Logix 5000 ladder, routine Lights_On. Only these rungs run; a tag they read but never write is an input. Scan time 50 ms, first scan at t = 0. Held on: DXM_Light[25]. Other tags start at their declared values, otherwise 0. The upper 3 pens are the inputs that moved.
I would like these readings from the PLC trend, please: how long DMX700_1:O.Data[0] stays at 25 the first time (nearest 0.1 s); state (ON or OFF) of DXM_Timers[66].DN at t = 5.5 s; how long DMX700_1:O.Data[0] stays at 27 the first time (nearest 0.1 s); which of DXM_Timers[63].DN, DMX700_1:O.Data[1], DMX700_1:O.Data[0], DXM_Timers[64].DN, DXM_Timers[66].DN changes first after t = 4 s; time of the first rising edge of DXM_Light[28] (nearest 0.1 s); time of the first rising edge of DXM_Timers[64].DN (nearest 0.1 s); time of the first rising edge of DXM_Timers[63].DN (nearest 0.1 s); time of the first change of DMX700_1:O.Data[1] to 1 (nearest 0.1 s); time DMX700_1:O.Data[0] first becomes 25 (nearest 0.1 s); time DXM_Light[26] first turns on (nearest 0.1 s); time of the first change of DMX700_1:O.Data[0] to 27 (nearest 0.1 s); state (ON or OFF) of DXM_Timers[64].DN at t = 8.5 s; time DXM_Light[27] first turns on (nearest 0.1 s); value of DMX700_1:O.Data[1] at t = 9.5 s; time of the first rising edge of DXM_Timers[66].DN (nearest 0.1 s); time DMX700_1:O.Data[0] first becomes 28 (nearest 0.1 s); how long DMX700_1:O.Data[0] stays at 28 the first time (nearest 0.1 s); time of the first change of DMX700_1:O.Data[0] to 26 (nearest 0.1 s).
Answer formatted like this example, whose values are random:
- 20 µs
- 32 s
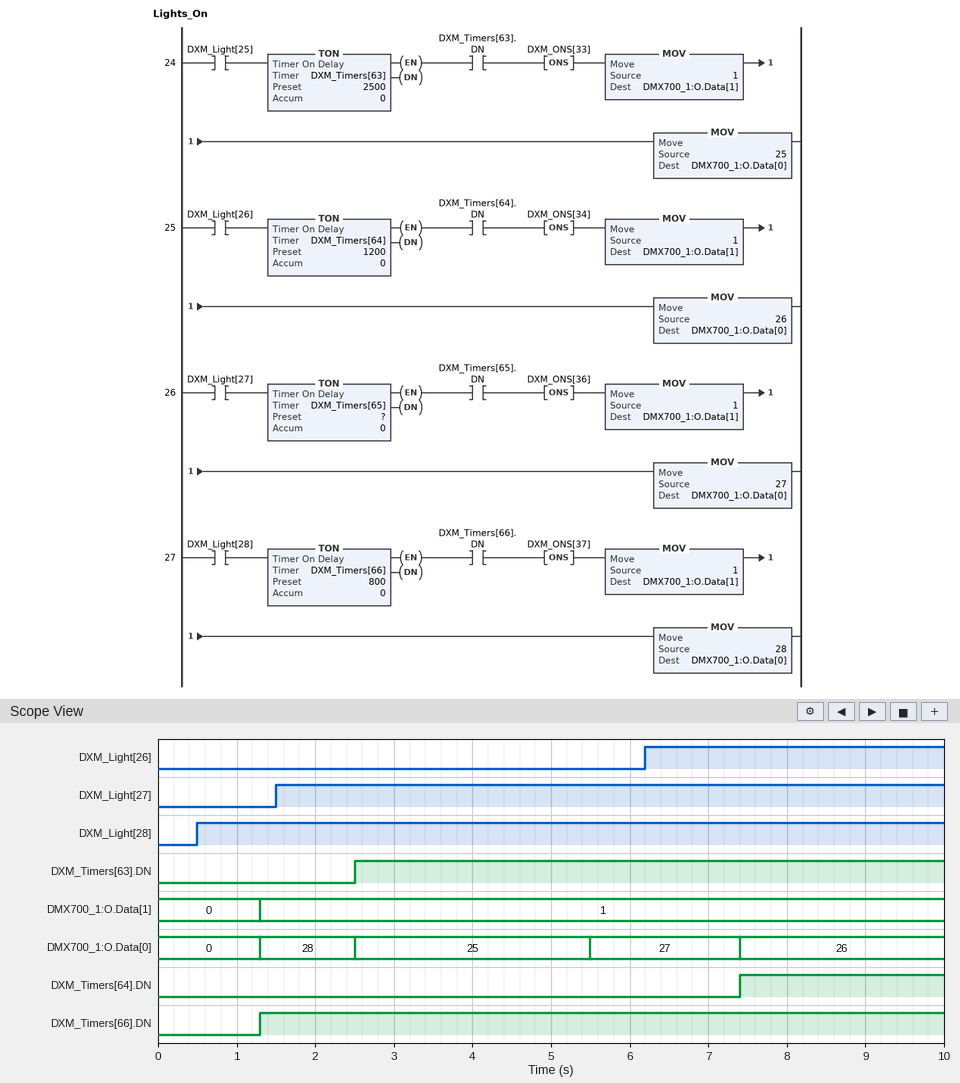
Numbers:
- 3.0 s
- ON
- 1.9 s
- DMX700_1:O.Data[0]
- 0.5 s
- 7.4 s
- 2.5 s
- 1.3 s
- 2.5 s
- 6.2 s
- 5.5 s
- ON
- 1.5 s
- 1
- 1.3 s
- 1.3 s
- 1.2 s
- 7.4 s
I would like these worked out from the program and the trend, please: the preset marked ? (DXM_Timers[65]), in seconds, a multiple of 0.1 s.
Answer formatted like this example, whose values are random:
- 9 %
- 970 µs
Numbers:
- 4.0 s
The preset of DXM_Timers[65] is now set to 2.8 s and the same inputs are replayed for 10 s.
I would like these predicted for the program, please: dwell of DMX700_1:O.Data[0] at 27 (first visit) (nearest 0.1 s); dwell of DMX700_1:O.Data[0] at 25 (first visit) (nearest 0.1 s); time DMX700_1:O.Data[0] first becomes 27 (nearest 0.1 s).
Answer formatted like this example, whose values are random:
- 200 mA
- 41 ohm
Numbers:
- 3.1 s
- 1.8 s
- 4.3 s
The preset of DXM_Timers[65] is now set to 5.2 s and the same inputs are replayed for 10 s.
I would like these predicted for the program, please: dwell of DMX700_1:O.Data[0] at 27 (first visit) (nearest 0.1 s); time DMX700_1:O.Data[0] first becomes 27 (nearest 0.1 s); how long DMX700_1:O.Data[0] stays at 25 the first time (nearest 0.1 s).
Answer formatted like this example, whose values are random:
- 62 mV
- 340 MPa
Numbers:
- 0.7 s
- 6.7 s
- 4.2 s
